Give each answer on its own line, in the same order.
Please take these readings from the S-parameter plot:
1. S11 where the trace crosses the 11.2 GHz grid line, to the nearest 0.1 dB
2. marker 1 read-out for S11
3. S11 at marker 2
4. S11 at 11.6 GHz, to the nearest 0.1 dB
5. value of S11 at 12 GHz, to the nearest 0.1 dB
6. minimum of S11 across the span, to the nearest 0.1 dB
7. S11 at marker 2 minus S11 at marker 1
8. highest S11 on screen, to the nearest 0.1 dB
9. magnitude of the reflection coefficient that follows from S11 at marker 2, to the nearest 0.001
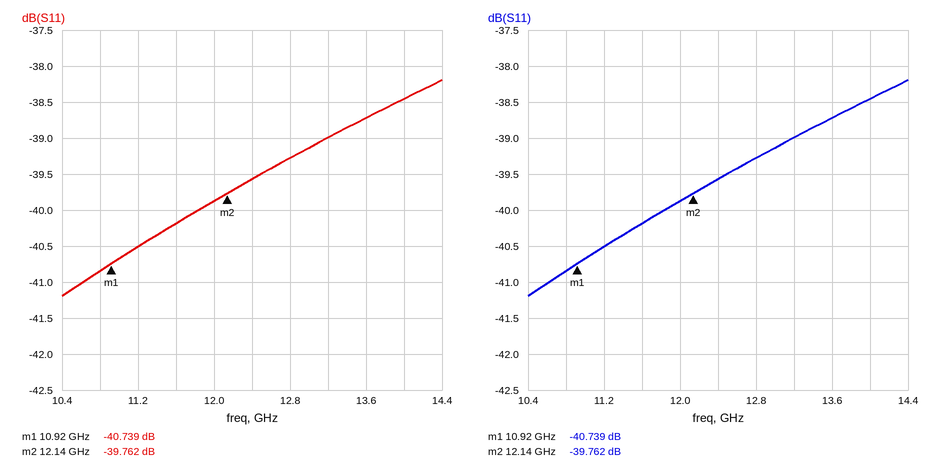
-40.5 dB
-40.739 dB
-39.762 dB
-40.2 dB
-39.9 dB
-41.2 dB
0.977 dB
-38.2 dB
0.010
